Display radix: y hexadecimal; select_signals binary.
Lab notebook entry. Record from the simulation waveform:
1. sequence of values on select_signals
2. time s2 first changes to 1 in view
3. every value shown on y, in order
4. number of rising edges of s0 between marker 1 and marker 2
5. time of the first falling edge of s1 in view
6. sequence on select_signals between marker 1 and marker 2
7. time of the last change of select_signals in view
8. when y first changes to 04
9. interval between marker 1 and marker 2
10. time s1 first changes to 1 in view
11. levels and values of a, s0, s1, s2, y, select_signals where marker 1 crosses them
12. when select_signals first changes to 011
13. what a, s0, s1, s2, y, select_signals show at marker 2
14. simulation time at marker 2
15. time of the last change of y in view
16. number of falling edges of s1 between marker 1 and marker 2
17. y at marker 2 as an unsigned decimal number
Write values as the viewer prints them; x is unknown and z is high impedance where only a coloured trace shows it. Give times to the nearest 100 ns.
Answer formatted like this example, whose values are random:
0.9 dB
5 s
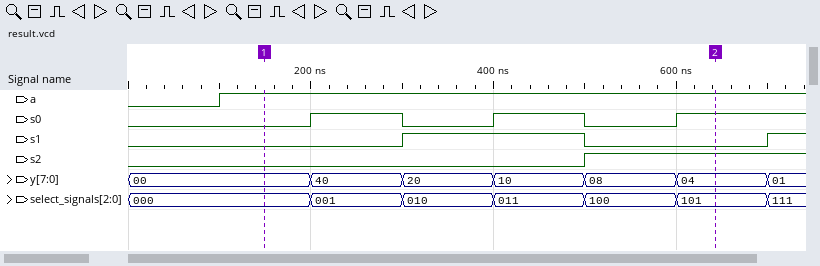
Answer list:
000, 001, 010, 011, 100, 101, 111
500 ns
00, 40, 20, 10, 08, 04, 01
3
500 ns
000, 001, 010, 011, 100, 101
700 ns
600 ns
500 ns
300 ns
a=1, s0=0, s1=0, s2=0, y=00, select_signals=000
400 ns
a=1, s0=1, s1=0, s2=1, y=04, select_signals=101
600 ns
700 ns
1
4
